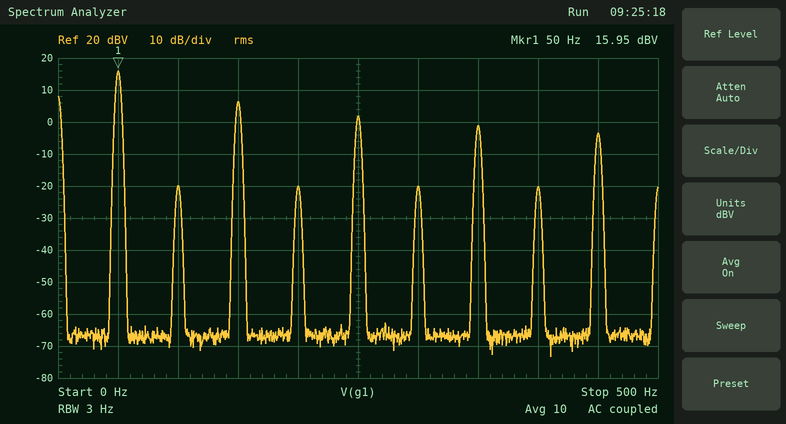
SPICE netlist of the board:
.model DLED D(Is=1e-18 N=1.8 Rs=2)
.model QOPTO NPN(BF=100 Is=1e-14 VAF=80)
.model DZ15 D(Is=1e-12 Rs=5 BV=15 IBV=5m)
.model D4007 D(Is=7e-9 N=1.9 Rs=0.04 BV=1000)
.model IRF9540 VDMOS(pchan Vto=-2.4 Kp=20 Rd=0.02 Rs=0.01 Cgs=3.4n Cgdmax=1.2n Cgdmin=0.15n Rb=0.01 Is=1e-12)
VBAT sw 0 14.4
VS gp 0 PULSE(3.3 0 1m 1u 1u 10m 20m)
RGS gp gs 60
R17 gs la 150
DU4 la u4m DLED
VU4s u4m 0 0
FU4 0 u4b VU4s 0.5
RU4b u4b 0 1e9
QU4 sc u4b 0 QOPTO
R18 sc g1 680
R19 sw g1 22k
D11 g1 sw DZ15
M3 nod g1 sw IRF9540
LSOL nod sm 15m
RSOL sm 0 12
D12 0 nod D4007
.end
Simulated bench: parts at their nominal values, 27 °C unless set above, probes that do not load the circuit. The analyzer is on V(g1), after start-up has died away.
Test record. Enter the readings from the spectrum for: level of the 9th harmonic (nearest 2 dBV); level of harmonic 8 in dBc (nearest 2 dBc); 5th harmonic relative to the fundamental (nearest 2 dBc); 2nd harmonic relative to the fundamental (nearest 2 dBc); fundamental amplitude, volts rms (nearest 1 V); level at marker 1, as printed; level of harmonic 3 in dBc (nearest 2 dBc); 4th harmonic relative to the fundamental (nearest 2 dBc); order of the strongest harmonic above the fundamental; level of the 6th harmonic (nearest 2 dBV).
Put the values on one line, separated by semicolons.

-4 dBV; -36 dBc; -14 dBc; -36 dBc; 6 V; 15.95 dBV; -10 dBc; -36 dBc; 3; -20 dBV
